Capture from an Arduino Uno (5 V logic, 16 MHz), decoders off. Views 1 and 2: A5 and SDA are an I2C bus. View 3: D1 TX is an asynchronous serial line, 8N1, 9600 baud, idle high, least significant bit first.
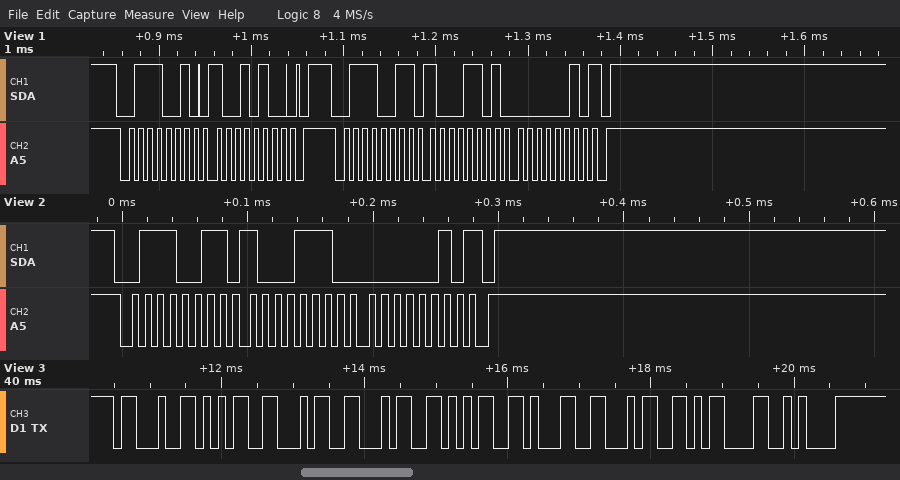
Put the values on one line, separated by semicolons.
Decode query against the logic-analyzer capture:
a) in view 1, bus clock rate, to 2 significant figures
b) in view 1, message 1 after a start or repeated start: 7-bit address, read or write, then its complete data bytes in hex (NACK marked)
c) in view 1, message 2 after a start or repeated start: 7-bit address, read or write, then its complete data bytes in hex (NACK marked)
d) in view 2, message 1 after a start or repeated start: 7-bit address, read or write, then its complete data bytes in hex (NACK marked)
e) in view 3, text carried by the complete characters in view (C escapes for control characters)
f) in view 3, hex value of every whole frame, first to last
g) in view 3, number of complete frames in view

100 kHz; 0x39 write: 94; 0x39 read: 8D 02 NACK; 0x39 read: 8E 02 NACK; "#544514\r\n"; 23 35 34 34 35 31 34 0D 0A; 9
